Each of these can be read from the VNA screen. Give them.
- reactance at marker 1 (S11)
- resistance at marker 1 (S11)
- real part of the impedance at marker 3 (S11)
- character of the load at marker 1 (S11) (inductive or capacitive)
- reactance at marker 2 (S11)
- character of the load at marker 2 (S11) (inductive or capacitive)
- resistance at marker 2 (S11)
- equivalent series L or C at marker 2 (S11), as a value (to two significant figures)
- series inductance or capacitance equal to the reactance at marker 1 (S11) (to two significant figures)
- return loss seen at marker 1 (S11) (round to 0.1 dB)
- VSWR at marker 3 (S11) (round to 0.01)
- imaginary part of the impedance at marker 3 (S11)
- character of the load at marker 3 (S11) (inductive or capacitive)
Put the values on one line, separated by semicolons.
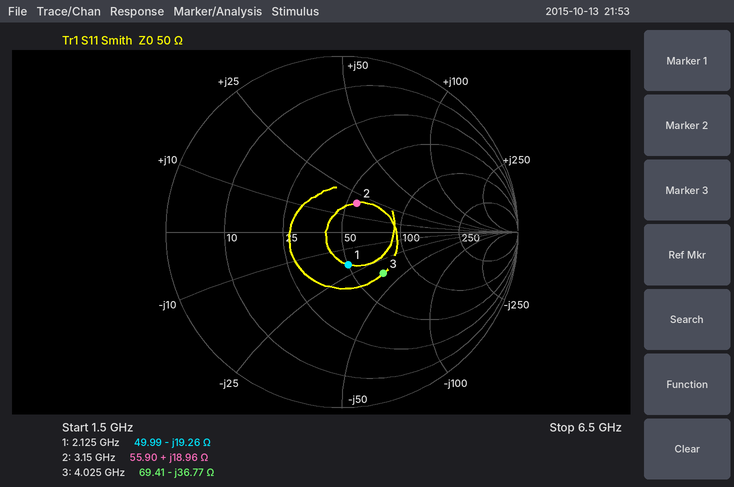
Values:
-19.26 Ω; 49.99 Ω; 69.41 Ω; capacitive; +18.96 Ω; inductive; 55.90 Ω; 960 pH; 3.9 pF; 14.5 dB; 2.00; -36.77 Ω; capacitive
